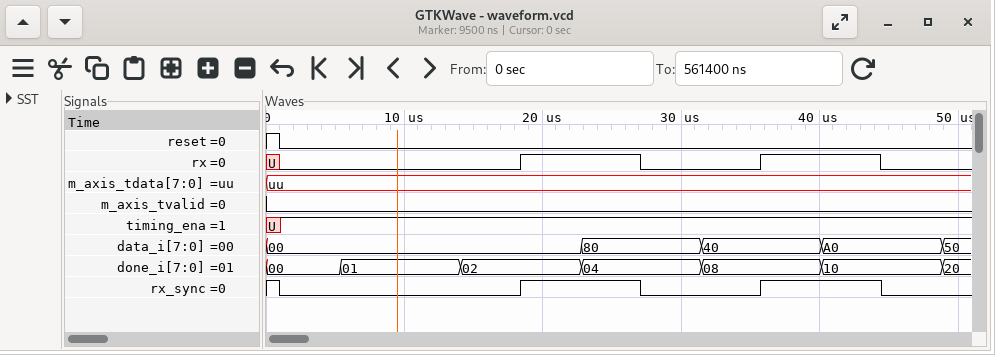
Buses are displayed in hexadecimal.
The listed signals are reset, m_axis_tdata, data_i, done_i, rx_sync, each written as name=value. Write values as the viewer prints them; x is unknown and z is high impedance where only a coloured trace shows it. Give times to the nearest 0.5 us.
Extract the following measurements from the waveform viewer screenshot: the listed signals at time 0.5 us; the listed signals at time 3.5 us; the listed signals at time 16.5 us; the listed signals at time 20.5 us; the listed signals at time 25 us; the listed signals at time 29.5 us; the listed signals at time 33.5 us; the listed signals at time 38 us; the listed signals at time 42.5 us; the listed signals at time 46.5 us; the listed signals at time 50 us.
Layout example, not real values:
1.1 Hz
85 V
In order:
reset=1, m_axis_tdata=uu, data_i=00, done_i=00, rx_sync=1
reset=0, m_axis_tdata=uu, data_i=00, done_i=00, rx_sync=0
reset=0, m_axis_tdata=uu, data_i=00, done_i=02, rx_sync=0
reset=0, m_axis_tdata=uu, data_i=00, done_i=02, rx_sync=1
reset=0, m_axis_tdata=uu, data_i=80, done_i=04, rx_sync=1
reset=0, m_axis_tdata=uu, data_i=80, done_i=04, rx_sync=0
reset=0, m_axis_tdata=uu, data_i=40, done_i=08, rx_sync=0
reset=0, m_axis_tdata=uu, data_i=40, done_i=08, rx_sync=1
reset=0, m_axis_tdata=uu, data_i=A0, done_i=10, rx_sync=1
reset=0, m_axis_tdata=uu, data_i=A0, done_i=10, rx_sync=0
reset=0, m_axis_tdata=uu, data_i=50, done_i=20, rx_sync=0
